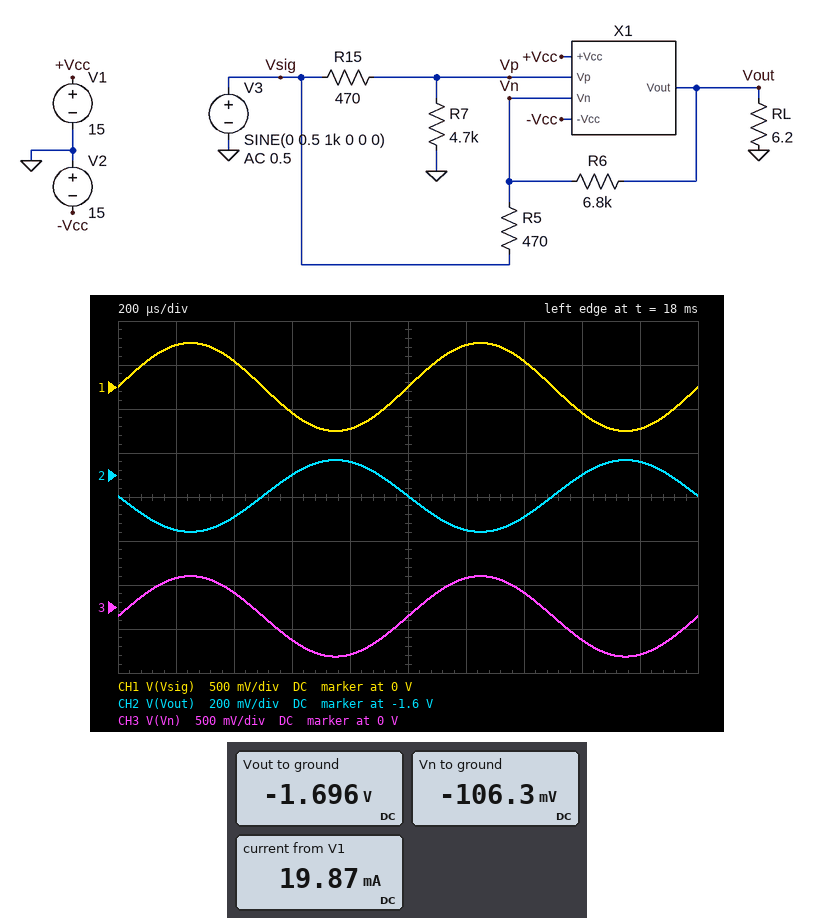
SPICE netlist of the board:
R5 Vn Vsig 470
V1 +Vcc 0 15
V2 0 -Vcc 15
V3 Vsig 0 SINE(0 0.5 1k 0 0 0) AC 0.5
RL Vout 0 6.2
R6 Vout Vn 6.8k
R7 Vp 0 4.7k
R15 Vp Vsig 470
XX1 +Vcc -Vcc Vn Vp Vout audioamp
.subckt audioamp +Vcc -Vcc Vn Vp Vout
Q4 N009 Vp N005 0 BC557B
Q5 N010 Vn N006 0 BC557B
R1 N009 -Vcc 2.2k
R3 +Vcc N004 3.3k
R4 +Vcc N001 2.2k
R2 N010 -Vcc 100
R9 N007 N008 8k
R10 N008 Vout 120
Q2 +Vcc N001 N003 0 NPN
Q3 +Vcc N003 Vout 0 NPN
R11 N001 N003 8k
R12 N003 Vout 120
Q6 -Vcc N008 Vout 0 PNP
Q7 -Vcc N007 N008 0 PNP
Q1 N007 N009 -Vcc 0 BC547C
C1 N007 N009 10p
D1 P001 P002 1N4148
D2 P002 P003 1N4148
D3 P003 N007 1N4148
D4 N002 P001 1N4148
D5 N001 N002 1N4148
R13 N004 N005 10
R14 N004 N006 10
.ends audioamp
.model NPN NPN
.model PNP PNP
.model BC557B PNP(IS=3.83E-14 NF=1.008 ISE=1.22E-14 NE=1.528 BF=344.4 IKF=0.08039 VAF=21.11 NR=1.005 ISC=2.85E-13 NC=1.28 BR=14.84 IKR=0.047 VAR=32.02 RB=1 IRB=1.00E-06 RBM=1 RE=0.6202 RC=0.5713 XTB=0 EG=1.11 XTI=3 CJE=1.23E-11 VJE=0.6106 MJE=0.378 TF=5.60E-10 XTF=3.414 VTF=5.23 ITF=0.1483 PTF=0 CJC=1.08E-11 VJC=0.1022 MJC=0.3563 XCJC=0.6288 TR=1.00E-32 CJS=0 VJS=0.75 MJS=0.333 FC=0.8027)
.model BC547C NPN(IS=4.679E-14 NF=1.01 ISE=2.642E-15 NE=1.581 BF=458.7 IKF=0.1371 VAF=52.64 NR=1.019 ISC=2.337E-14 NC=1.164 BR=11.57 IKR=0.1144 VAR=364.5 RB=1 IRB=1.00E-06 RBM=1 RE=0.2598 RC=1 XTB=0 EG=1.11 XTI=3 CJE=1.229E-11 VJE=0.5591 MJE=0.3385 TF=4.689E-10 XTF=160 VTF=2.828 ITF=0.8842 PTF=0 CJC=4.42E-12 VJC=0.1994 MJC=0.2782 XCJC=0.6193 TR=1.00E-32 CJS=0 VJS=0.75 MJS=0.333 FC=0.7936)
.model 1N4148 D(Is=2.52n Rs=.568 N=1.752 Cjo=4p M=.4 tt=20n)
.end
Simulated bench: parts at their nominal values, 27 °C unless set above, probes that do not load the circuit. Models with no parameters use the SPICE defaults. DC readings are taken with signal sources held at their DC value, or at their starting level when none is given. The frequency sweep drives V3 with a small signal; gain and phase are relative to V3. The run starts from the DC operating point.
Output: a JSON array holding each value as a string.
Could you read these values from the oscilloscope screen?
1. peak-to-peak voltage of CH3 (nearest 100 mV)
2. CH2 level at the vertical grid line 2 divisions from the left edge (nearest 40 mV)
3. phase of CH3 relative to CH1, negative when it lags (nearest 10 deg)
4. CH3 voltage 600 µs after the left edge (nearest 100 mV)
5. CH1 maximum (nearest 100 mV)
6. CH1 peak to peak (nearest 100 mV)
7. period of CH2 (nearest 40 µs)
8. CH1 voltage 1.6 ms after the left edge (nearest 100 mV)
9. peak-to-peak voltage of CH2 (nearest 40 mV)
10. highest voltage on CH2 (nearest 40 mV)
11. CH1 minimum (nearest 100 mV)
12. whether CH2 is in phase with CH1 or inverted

["900 mV", "-1.80 V", "0 deg", "-400 mV", "500 mV", "1.0 V", "1.00 ms", "-300 mV", "320 mV", "-1.52 V", "-500 mV", "inverted"]
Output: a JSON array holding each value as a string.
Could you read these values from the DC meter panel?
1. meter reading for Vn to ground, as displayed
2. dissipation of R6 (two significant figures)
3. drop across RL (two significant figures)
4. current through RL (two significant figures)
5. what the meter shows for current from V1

["-106.3 mV", "370 µW", "1.7 V", "270 mA", "19.87 mA"]
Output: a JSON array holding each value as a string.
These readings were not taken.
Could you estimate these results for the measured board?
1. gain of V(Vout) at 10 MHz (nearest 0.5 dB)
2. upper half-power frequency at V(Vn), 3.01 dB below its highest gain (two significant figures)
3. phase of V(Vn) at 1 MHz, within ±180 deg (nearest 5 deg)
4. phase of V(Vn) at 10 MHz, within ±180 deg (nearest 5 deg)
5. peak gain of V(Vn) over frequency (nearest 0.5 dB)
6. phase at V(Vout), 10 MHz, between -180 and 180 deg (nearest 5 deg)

["-20.0 dB", "160 MHz", "0 deg", "-5 deg", "-0.5 dB", "95 deg"]
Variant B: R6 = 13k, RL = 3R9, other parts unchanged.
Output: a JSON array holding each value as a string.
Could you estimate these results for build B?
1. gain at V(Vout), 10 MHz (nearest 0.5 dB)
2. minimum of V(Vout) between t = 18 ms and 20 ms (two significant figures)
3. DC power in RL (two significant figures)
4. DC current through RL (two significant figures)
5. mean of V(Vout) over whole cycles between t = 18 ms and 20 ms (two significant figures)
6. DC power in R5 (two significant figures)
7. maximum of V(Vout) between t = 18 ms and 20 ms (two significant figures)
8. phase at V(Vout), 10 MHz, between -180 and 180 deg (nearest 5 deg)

["-8.5 dB", "-3.9 V", "2.5 W", "800 mA", "-3.1 V", "24 µW", "-2.4 V", "55 deg"]
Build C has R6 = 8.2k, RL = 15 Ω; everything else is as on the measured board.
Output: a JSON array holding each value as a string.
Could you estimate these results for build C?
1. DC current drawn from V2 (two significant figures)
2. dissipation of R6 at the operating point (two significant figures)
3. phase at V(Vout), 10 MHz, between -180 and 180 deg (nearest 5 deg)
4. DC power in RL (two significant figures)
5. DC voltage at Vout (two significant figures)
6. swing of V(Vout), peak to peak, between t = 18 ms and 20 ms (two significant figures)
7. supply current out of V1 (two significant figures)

["160 mA", "450 µW", "75 deg", "270 mW", "-2.0 V", "580 mV", "24 mA"]
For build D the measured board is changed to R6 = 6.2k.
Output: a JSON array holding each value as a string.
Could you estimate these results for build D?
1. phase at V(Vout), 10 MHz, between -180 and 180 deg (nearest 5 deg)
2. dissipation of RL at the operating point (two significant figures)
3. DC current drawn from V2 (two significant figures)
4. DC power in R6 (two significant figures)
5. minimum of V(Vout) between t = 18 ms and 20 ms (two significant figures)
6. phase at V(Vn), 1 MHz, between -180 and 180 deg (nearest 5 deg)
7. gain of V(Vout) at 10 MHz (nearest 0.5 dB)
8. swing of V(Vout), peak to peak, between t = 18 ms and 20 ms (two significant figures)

["140 deg", "390 mW", "270 mA", "340 µW", "-1.7 V", "0 deg", "-25.5 dB", "220 mV"]
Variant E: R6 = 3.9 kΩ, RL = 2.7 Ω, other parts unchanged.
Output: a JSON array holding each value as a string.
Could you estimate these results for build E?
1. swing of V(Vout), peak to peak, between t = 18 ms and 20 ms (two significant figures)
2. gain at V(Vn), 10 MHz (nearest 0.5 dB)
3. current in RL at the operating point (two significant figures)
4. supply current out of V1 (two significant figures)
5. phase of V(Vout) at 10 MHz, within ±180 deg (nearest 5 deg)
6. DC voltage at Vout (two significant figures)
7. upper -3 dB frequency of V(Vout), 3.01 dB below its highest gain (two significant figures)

["200 mV", "-1.0 dB", "380 mA", "18 mA", "-90 deg", "-1.0 V", "16 MHz"]
